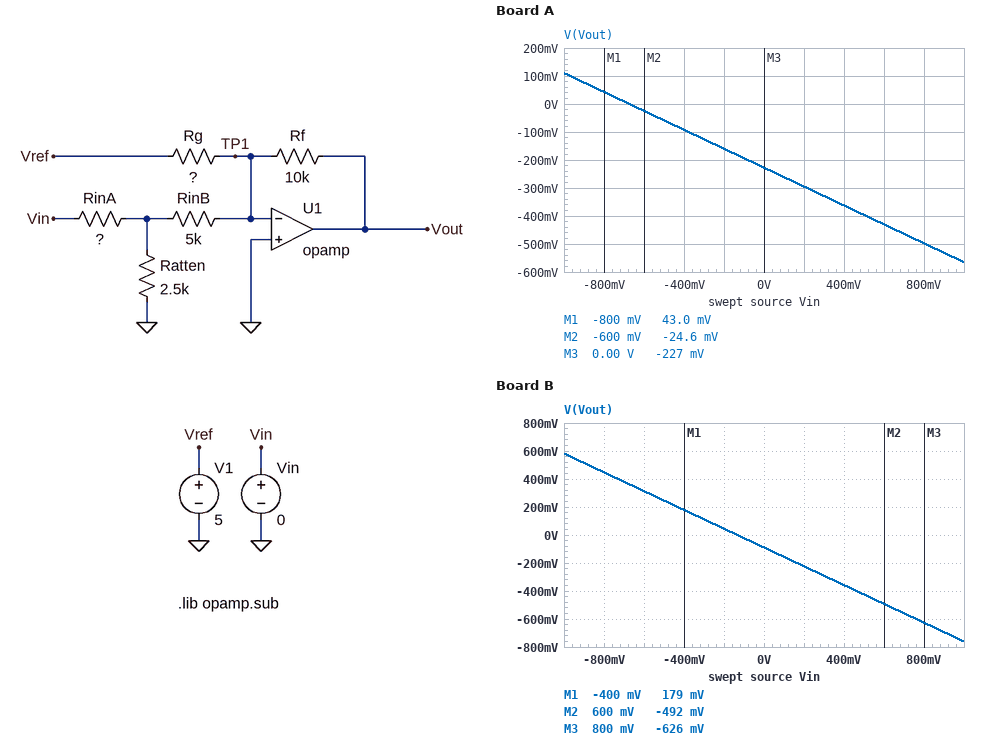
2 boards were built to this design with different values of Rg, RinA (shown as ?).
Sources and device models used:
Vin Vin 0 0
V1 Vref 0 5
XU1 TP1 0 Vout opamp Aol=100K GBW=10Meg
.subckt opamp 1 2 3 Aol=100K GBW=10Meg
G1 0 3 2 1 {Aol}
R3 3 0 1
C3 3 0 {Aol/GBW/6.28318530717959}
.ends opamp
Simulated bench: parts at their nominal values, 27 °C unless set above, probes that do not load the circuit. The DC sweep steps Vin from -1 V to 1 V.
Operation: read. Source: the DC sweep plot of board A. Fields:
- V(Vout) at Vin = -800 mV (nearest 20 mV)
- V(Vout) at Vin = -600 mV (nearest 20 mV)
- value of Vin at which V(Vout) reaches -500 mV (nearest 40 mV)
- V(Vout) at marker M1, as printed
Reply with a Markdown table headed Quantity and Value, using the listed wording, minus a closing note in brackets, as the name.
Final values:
| Quantity | Value |
|---|---|
| V(Vout) at Vin = -800 mV | 40 mV |
| V(Vout) at Vin = -600 mV | -20 mV |
| value of Vin at which V(Vout) reaches -500 mV | 800 mV |
| V(Vout) at marker M1, as printed | 43.0 mV |
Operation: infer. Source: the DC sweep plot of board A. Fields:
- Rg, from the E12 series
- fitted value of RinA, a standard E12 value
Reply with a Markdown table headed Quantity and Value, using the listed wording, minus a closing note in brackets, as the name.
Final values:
| Quantity | Value |
|---|---|
| Rg, from the E12 series | 220 kΩ |
| fitted value of RinA, a standard E12 value | 8.2 kΩ |
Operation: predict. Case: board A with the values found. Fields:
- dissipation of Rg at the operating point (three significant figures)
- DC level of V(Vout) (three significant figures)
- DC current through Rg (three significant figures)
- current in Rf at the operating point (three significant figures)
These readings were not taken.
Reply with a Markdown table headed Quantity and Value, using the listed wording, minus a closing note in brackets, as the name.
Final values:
| Quantity | Value |
|---|---|
| dissipation of Rg at the operating point | 114 µW |
| DC level of V(Vout) | -227 mV |
| DC current through Rg | 22.7 µA |
| current in Rf at the operating point | 22.7 µA |
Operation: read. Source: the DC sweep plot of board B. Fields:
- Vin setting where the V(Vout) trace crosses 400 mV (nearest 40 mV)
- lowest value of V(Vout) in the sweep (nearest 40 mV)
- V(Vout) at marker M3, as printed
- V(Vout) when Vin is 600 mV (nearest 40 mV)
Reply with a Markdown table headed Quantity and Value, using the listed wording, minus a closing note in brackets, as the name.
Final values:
| Quantity | Value |
|---|---|
| Vin setting where the V(Vout) trace crosses 400 mV | -720 mV |
| lowest value of V(Vout) in the sweep | -760 mV |
| V(Vout) at marker M3, as printed | -626 mV |
| V(Vout) when Vin is 600 mV | -480 mV |
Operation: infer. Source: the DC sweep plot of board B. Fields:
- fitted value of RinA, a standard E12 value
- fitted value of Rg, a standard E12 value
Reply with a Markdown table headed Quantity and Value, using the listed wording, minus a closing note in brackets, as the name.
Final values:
| Quantity | Value |
|---|---|
| fitted value of RinA, a standard E12 value | 3.3 kΩ |
| fitted value of Rg, a standard E12 value | 560 kΩ |
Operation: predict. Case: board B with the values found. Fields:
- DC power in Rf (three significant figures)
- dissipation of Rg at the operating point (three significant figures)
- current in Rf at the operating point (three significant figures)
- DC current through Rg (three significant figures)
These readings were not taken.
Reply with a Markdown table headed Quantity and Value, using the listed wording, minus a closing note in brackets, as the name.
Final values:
| Quantity | Value |
|---|---|
| DC power in Rf | 797 nW |
| dissipation of Rg at the operating point | 44.6 µW |
| current in Rf at the operating point | 8.93 µA |
| DC current through Rg | 8.93 µA |
